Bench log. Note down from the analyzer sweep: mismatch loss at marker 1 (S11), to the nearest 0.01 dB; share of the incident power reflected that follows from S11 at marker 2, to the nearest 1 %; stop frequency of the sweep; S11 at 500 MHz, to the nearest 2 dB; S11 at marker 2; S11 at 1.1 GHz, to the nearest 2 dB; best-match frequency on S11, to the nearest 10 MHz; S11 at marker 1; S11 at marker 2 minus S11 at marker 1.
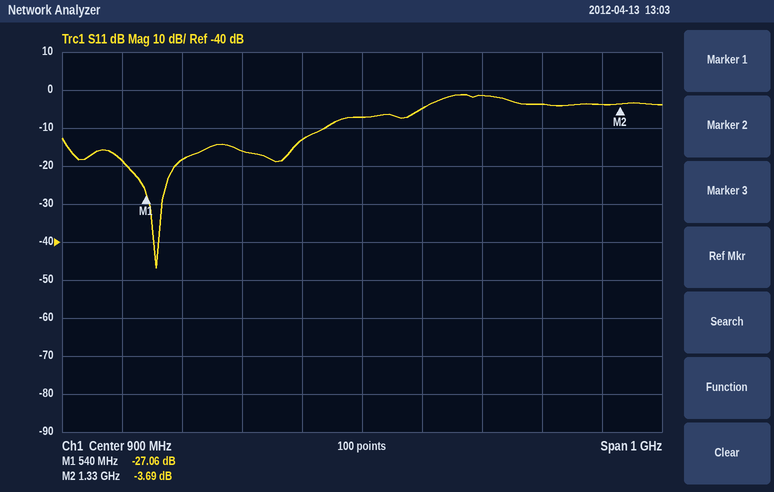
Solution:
0.01 dB
43 %
1.4 GHz
-18 dB
-3.69 dB
-2 dB
560 MHz
-27.06 dB
23.37 dB
